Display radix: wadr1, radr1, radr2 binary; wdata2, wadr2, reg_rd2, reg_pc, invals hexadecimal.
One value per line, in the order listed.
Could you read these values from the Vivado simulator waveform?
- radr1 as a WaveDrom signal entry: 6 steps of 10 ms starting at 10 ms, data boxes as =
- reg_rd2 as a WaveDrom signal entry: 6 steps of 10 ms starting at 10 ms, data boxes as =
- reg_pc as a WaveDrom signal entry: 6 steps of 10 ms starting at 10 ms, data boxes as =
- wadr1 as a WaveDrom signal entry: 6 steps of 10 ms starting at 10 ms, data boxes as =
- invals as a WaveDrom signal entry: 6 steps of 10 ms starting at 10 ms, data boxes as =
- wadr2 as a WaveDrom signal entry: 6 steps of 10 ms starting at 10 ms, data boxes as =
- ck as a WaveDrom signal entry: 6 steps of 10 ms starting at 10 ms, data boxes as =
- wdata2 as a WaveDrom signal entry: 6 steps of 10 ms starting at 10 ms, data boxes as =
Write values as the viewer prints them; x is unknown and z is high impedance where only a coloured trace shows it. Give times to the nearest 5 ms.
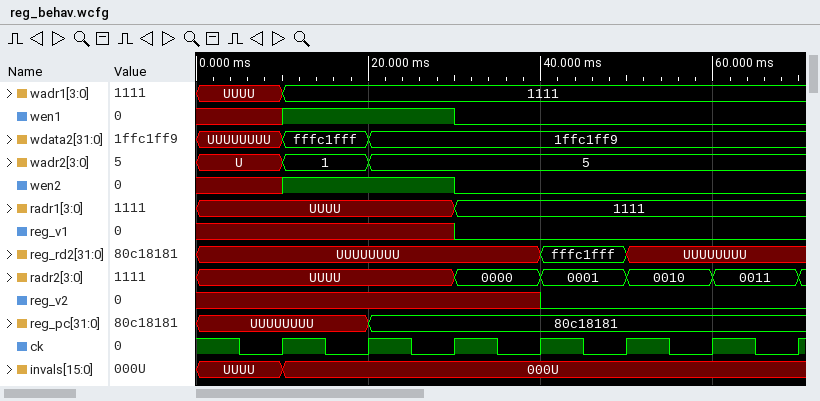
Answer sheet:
{name: 'radr1', wave: 'x.=...', data: '1111'}
{name: 'reg_rd2', wave: 'x..=x.', data: 'fffc1fff'}
{name: 'reg_pc', wave: 'x=....', data: '80c18181'}
{name: 'wadr1', wave: '=.....', data: '1111'}
{name: 'invals', wave: '=.....', data: '000U'}
{name: 'wadr2', wave: '==....', data: '1 5'}
{name: 'ck', wave: 'p.....'}
{name: 'wdata2', wave: '==....', data: 'fffc1fff 1ffc1ff9'}
